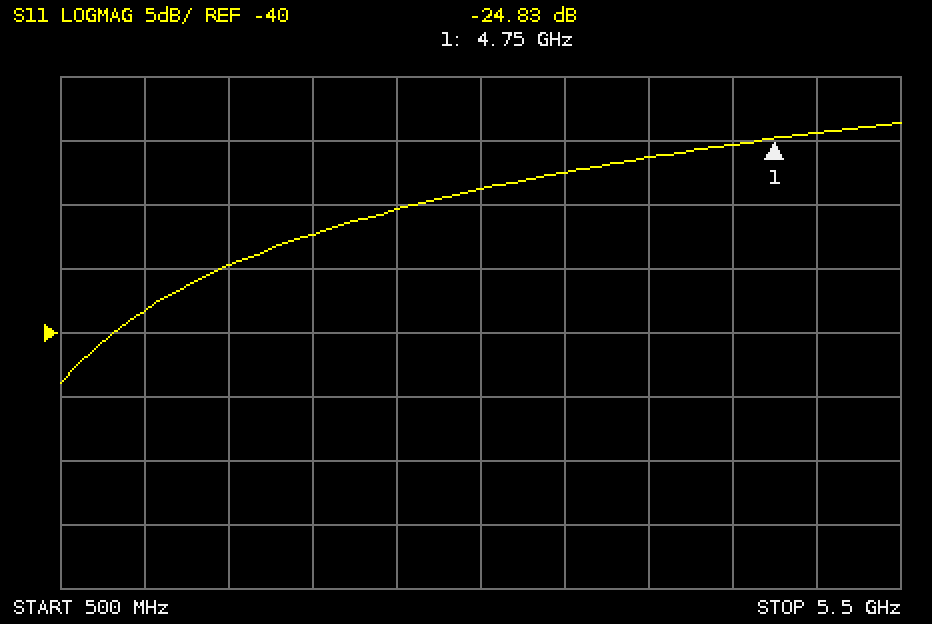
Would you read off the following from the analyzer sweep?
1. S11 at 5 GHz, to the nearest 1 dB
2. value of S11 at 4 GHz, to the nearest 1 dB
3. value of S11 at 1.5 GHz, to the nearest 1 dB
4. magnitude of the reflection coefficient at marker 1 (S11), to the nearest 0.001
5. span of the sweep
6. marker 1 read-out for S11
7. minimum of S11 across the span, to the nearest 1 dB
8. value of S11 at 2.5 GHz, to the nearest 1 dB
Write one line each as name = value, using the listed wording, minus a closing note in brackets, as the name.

S11 at 5 GHz, to the nearest 1 dB = -24 dB
value of S11 at 4 GHz, to the nearest 1 dB = -26 dB
value of S11 at 1.5 GHz, to the nearest 1 dB = -35 dB
magnitude of the reflection coefficient at marker 1 (S11), to the nearest 0.001 = 0.057
span of the sweep = 5 GHz
marker 1 read-out for S11 = -24.83 dB
minimum of S11 across the span, to the nearest 1 dB = -44 dB
value of S11 at 2.5 GHz, to the nearest 1 dB = -30 dB
